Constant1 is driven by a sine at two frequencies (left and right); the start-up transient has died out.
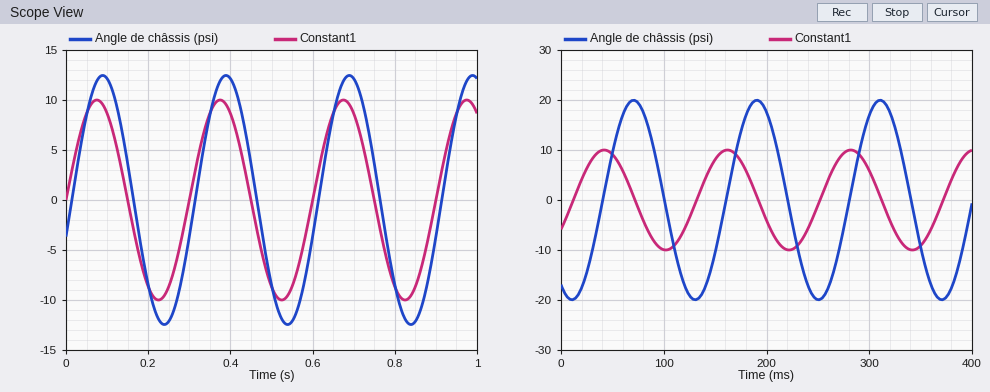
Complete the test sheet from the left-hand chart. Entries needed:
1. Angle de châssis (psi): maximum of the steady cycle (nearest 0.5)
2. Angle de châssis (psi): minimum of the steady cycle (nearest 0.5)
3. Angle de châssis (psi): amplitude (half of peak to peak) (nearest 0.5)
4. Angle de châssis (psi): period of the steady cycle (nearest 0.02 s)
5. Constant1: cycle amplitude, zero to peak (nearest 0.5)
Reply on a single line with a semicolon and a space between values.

12.5; -12.5; 12.5; 0.30 s; 10.0
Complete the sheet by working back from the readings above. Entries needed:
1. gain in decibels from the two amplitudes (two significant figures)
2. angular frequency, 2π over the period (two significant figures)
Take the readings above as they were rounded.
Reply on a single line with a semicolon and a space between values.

1.9 dB; 21 rad/s
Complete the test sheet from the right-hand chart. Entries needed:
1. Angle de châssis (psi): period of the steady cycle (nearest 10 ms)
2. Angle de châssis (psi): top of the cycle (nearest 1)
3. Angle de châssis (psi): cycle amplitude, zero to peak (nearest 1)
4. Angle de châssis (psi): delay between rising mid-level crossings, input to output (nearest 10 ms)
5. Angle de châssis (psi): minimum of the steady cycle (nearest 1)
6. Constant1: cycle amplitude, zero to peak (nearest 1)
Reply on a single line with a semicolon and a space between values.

120 ms; 20; 20; 30 ms; -20; 10
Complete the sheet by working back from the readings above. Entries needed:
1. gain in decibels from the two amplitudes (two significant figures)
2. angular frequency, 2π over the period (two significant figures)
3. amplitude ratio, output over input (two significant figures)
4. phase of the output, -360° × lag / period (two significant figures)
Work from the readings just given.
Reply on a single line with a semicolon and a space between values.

6.0 dB; 0.052 rad/ms; 2.0; -90°
